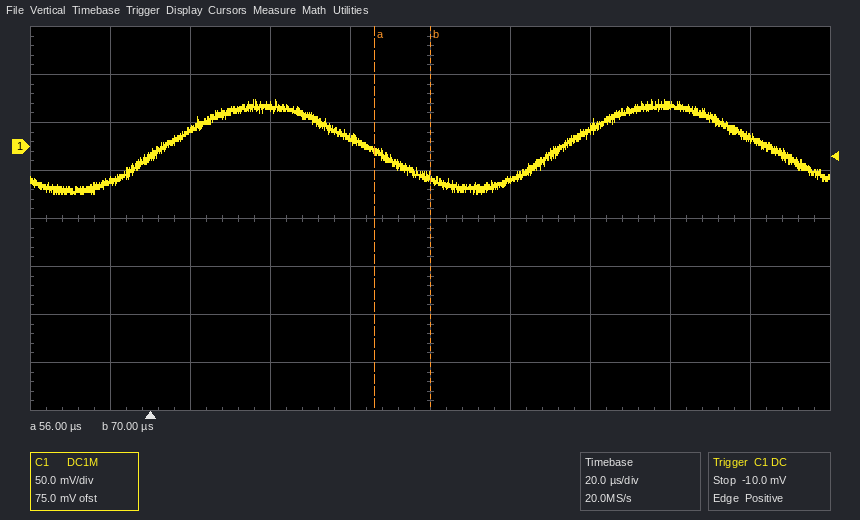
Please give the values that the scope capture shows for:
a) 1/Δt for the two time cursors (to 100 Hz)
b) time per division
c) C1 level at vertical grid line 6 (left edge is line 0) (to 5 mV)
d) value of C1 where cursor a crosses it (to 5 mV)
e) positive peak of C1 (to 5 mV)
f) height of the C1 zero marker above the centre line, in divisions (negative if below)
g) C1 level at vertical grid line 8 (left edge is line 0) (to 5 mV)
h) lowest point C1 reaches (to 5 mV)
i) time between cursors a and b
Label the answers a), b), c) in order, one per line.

a) 71.4 kHz
b) 20 µs
c) -35 mV
d) -5 mV
e) 50 mV
f) +1.5 div
g) 45 mV
h) -50 mV
i) 14 µs
